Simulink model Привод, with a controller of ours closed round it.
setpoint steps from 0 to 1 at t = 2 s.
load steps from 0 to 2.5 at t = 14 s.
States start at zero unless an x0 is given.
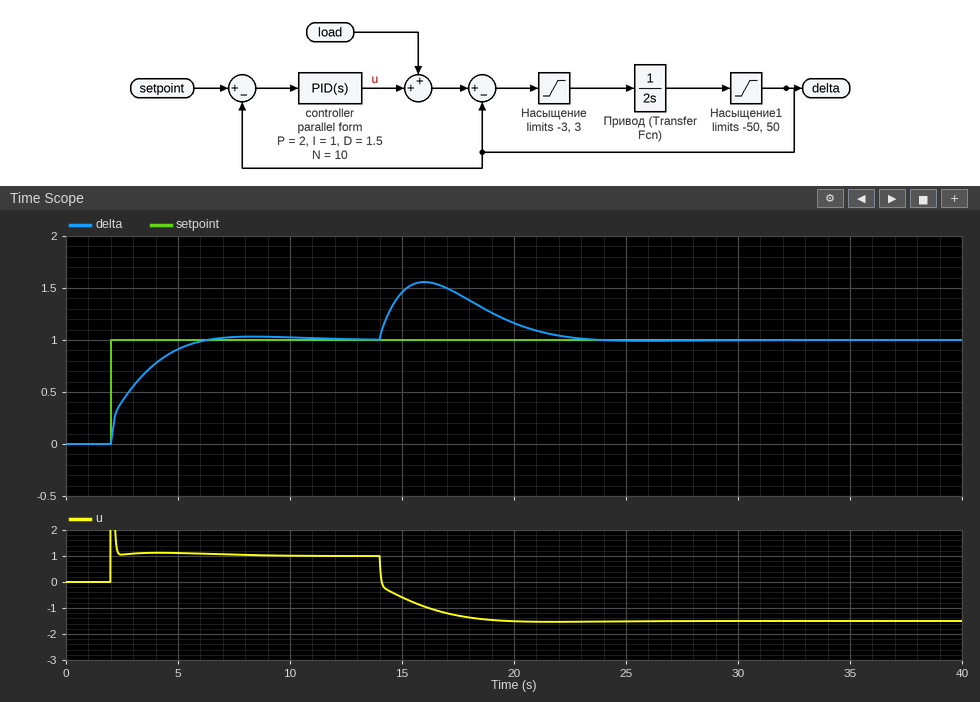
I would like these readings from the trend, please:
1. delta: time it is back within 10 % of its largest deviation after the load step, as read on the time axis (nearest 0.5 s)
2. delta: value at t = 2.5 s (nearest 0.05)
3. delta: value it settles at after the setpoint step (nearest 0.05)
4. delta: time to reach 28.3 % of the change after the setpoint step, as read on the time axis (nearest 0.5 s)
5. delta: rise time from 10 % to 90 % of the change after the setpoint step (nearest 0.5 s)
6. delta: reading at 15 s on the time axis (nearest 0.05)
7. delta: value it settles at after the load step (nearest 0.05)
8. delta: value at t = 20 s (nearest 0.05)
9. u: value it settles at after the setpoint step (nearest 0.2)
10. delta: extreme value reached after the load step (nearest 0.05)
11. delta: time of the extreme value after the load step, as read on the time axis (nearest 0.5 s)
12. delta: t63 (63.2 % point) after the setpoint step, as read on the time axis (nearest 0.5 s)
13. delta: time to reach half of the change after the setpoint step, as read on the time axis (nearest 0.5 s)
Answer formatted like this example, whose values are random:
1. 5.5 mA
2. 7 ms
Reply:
1. 21.5 s
2. 0.40
3. 1.00
4. 2.0 s
5. 3.0 s
6. 1.45
7. 1.00
8. 1.15
9. 1.0
10. 1.55
11. 16.0 s
12. 3.5 s
13. 3.0 s
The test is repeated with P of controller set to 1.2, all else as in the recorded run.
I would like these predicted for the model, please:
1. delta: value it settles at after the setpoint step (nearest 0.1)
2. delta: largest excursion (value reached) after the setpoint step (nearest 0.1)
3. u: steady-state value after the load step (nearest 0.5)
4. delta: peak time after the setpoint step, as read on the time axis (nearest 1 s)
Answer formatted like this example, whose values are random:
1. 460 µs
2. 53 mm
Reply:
1. 1.0
2. 1.1
3. -1.5
4. 8 s
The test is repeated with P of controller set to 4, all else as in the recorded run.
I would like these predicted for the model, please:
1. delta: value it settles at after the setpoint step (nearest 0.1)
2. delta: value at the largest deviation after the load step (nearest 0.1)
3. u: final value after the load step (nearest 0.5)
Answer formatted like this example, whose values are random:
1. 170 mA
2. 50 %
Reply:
1. 1.0
2. 1.4
3. -1.5
